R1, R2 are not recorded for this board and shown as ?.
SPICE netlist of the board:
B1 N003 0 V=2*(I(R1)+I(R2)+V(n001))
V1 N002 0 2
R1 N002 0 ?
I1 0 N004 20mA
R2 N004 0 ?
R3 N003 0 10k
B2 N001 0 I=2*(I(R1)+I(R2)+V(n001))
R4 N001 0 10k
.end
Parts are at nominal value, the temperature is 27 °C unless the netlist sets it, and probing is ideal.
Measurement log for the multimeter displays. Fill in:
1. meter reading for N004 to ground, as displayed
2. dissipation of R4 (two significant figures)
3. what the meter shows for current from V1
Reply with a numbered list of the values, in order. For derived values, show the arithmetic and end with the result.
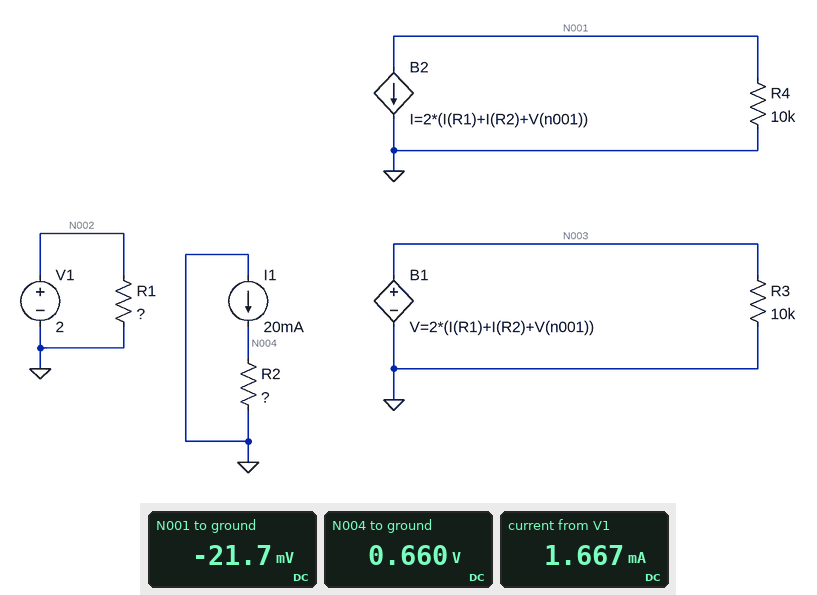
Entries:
1. 0.660 V
2. (0 V - (-21.7 mV))^2 / 10 kΩ = 47 nW
3. 1.667 mA
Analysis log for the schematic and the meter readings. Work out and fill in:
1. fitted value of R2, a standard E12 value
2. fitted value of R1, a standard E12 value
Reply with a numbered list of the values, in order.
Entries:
1. 33 Ω
2. 1.2 kΩ
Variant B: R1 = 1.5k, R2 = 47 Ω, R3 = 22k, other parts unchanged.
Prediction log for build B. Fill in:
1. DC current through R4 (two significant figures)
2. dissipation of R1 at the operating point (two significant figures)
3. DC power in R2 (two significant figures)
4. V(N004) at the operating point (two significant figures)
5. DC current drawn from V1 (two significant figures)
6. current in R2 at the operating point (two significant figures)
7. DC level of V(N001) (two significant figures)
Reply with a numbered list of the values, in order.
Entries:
1. 2.1 µA
2. 2.7 mW
3. 19 mW
4. 940 mV
5. 1.3 mA
6. 20 mA
7. -21 mV
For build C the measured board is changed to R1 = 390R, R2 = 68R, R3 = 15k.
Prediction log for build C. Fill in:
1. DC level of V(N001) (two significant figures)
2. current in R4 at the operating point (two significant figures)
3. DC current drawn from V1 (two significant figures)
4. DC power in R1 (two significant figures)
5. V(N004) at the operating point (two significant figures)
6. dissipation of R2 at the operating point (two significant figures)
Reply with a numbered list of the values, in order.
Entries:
1. -25 mV
2. 2.5 µA
3. 5.1 mA
4. 10 mW
5. 1.4 V
6. 27 mW
